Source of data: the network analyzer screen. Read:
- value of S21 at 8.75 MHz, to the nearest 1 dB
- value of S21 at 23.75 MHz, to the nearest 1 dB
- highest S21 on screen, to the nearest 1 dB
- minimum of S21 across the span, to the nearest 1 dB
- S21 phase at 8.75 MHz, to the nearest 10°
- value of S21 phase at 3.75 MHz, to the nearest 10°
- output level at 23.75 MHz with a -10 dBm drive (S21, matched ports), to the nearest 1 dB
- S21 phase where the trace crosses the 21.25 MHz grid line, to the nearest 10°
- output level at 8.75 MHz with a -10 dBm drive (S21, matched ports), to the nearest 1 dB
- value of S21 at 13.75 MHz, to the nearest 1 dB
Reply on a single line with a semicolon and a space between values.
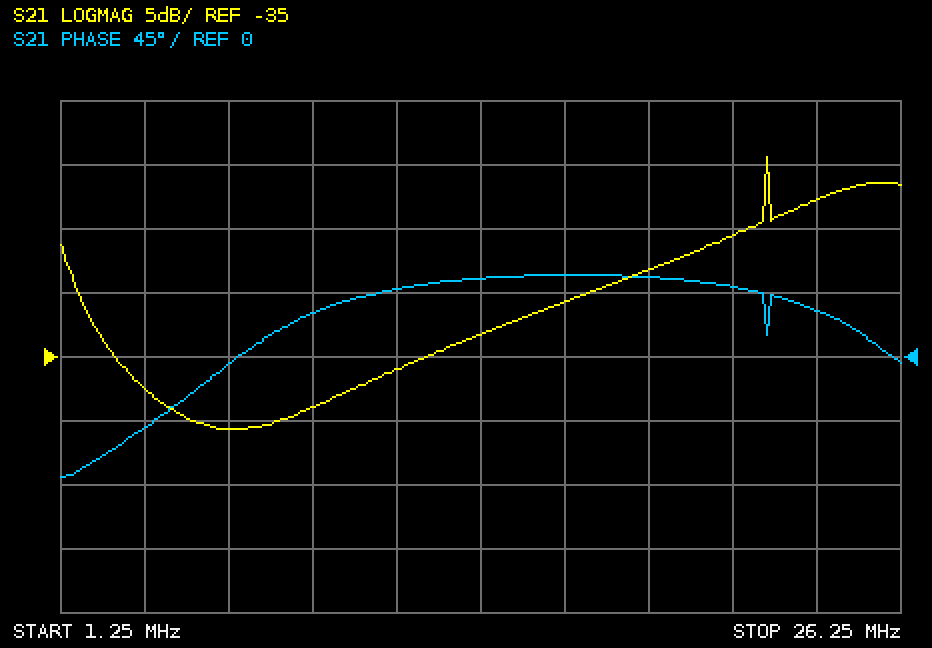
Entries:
-39 dB; -23 dB; -19 dB; -41 dB; 30°; -50°; -33 dBm; 50°; -49 dBm; -33 dB
